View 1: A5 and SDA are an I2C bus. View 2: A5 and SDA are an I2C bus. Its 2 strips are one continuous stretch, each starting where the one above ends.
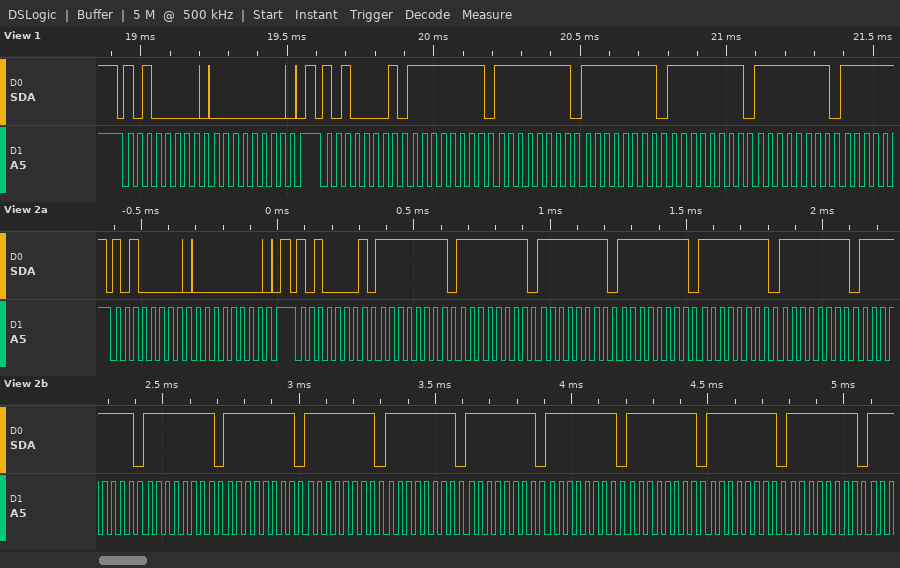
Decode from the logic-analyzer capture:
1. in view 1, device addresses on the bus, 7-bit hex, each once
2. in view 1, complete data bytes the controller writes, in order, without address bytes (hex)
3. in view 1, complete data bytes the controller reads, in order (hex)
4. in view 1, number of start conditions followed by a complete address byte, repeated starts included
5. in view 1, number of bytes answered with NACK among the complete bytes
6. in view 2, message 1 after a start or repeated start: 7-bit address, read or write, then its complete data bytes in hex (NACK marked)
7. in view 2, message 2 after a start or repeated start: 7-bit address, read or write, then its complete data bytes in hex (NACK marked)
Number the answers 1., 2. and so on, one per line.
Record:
1. 0x50
2. 00
3. FF FF FF FF FF
4. 2
5. 0
6. 0x50 write: 00
7. 0x50 read: FF FF FF FF FF FF FF FF FF FF FF FF FF FF FF FF
